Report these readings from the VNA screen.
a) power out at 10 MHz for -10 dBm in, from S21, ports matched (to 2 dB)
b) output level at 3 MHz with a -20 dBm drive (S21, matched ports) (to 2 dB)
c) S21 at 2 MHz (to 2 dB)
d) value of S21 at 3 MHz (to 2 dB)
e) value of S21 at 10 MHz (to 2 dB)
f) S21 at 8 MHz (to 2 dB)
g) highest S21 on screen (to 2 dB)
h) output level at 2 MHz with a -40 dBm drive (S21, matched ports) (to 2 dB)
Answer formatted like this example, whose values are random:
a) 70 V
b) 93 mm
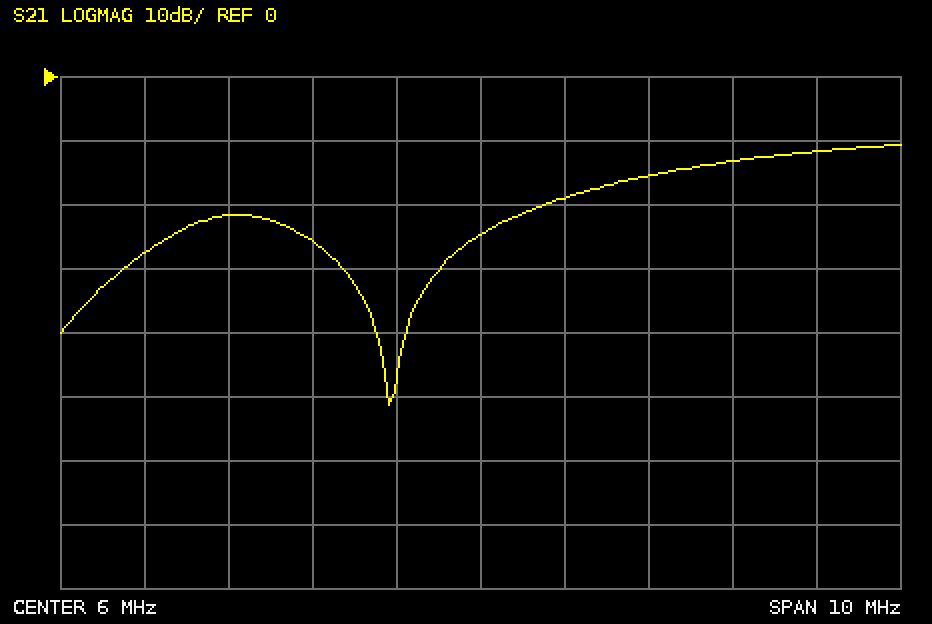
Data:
a) -22 dBm
b) -42 dBm
c) -28 dB
d) -22 dB
e) -12 dB
f) -16 dB
g) -10 dB
h) -68 dBm
